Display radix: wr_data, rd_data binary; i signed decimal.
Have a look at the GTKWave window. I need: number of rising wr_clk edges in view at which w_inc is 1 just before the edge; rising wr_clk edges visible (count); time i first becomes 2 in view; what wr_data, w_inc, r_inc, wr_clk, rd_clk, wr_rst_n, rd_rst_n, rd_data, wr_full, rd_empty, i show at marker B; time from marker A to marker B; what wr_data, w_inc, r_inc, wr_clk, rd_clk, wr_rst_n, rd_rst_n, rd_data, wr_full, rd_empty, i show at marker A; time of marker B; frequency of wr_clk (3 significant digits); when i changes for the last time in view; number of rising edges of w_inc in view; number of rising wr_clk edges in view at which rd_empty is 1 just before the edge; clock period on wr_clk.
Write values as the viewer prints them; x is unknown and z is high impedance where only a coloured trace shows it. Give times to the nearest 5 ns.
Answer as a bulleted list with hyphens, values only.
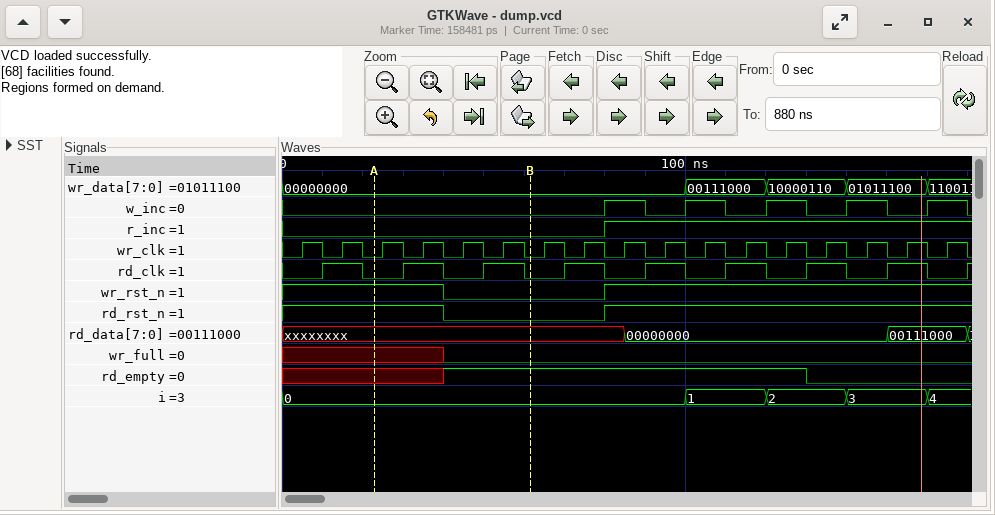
- 5
- 17
- 120 ns
- wr_data=00000000, w_inc=0, r_inc=0, wr_clk=0, rd_clk=0, wr_rst_n=0, rd_rst_n=0, rd_data=xxxxxxxx, wr_full=0, rd_empty=1, i=0
- 40 ns
- wr_data=00000000, w_inc=0, r_inc=0, wr_clk=0, rd_clk=0, wr_rst_n=1, rd_rst_n=1, rd_data=xxxxxxxx, wr_full=x, rd_empty=x, i=0
- 60 ns
- 100 MHz
- 160 ns
- 5
- 9
- 10 ns
